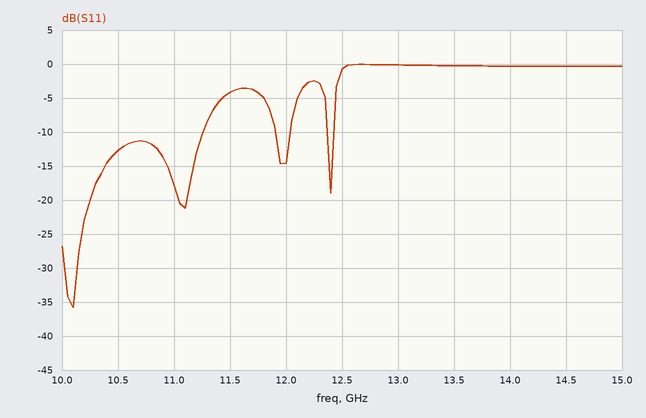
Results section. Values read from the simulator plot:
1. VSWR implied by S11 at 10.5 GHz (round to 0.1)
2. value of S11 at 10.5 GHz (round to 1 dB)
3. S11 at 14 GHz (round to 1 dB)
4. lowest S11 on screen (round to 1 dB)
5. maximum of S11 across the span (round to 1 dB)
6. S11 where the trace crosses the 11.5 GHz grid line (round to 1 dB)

1.6
-13 dB
0 dB
-36 dB
0 dB
-4 dB
